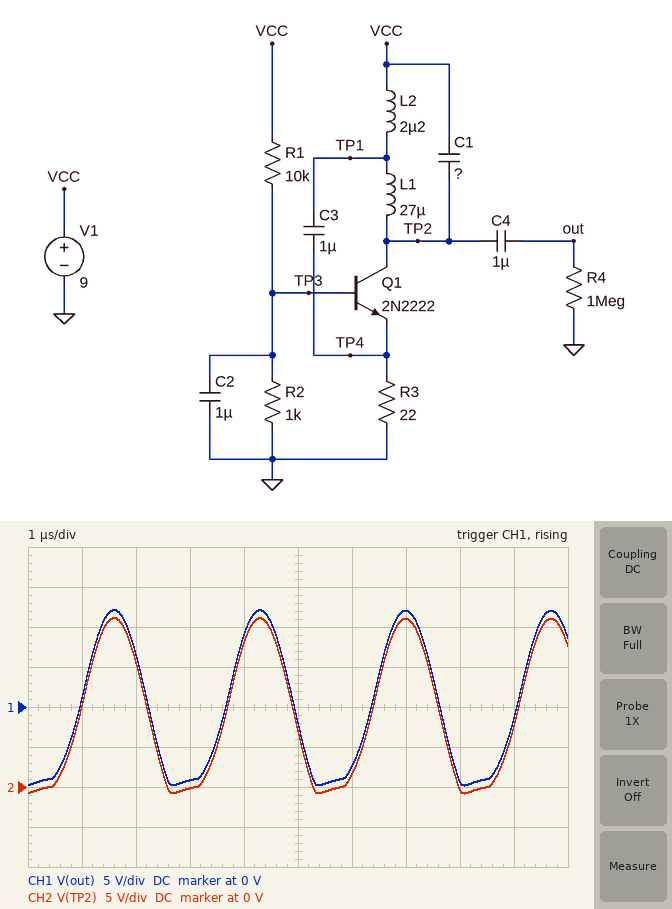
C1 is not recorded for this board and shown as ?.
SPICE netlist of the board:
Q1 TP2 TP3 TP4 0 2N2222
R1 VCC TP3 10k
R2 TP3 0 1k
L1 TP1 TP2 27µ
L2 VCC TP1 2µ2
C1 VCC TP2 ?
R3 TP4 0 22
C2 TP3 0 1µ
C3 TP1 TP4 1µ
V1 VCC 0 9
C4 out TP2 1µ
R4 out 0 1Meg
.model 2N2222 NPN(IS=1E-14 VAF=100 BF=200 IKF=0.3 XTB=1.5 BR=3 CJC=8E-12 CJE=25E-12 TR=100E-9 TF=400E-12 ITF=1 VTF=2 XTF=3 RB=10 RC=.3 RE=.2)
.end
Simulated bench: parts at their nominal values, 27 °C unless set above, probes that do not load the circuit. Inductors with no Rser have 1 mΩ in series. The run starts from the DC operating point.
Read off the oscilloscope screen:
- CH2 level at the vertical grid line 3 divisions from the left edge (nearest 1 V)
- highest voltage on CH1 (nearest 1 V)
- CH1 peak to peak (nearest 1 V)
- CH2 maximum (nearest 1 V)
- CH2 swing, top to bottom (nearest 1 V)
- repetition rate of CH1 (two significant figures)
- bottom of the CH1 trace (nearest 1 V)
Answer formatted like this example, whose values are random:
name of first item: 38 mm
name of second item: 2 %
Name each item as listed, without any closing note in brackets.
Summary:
CH2 level at the vertical grid line 3 divisions from the left edge: 0 V
highest voltage on CH1: 12 V
CH1 peak to peak: 22 V
CH2 maximum: 21 V
CH2 swing, top to bottom: 22 V
repetition rate of CH1: 370 kHz
bottom of the CH1 trace: -10 V
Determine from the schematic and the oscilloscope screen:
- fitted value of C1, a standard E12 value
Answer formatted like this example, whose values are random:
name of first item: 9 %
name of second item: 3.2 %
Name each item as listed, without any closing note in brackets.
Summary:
fitted value of C1, a standard E12 value: 5.6 nF
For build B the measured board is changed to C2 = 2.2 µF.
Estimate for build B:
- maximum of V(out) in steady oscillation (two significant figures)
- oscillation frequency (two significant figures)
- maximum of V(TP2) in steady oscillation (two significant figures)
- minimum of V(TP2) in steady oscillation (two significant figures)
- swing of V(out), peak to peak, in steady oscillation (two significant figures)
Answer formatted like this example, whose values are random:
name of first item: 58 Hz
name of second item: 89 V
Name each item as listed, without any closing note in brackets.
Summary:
maximum of V(out) in steady oscillation: 13 V
oscillation frequency: 360 kHz
maximum of V(TP2) in steady oscillation: 22 V
minimum of V(TP2) in steady oscillation: -810 mV
swing of V(out), peak to peak, in steady oscillation: 23 V
